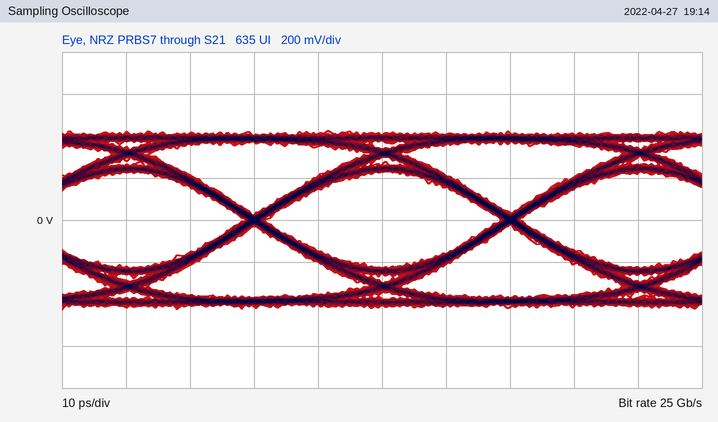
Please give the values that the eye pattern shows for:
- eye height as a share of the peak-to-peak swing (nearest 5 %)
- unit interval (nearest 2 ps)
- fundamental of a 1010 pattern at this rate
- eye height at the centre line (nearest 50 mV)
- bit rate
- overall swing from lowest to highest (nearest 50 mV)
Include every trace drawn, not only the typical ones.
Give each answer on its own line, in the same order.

55 %
40 ps
12.5 GHz
450 mV
25 Gb/s
850 mV
